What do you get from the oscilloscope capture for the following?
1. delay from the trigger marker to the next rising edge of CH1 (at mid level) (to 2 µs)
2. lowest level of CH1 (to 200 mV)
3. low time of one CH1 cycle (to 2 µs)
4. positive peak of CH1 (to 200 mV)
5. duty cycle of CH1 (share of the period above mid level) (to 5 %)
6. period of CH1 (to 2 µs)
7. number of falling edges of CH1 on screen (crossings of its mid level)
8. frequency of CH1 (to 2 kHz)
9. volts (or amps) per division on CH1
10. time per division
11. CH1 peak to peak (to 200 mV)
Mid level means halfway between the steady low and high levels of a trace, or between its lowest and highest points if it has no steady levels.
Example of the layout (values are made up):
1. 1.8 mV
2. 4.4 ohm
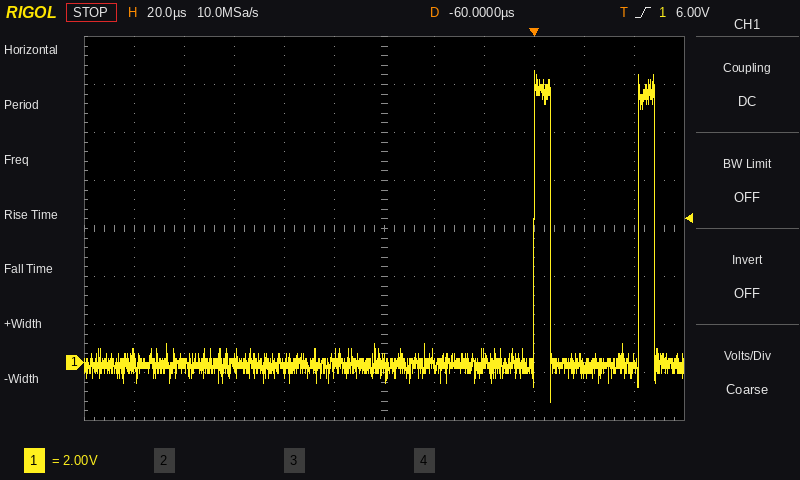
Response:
1. 42 µs
2. -1.6 V
3. 36 µs
4. 12.2 V
5. 15 %
6. 42 µs
7. 2
8. 24 kHz
9. 2 V
10. 20 µs
11. 13.8 V
